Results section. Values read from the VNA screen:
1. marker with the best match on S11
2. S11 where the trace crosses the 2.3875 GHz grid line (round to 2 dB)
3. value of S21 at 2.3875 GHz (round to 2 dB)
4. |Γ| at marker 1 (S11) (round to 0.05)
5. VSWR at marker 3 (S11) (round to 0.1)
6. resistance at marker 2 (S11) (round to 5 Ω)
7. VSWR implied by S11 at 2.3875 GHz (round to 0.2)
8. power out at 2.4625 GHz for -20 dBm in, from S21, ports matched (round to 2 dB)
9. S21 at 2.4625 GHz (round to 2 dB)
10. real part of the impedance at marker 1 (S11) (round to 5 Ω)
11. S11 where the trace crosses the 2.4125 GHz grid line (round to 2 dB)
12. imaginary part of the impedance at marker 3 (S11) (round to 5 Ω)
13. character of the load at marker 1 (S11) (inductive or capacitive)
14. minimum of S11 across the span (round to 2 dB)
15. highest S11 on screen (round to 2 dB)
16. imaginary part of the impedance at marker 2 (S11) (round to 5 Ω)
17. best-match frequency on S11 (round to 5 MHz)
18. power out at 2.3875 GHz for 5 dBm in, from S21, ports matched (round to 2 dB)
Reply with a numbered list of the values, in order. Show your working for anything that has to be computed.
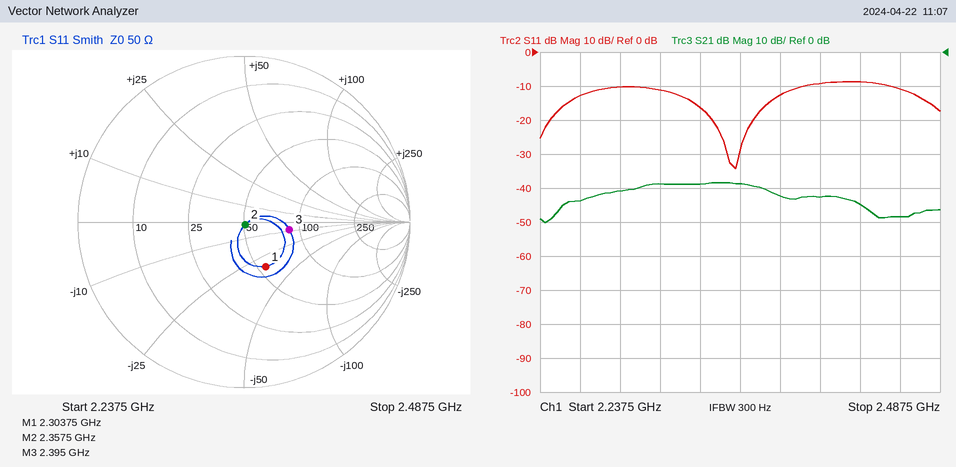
1. marker 2
2. -12 dB
3. -42 dB
4. 0.30
5. 1.8
6. 50 Ω
7. |Γ| = 10^(-12/20) = 0.2512; VSWR = (1 + 0.2512)/(1 − 0.2512) ≈ 1.67, so 1.6 to the nearest 0.2
8. -20 dBm + (-48 dB) = -68 dBm
9. -48 dB
10. 55 Ω
11. -10 dB
12. -10 Ω
13. capacitive
14. -34 dB
15. -8 dB
16. 0 Ω
17. 2.360 GHz
18. 5 dBm + (-42 dB) = -38 dBm
